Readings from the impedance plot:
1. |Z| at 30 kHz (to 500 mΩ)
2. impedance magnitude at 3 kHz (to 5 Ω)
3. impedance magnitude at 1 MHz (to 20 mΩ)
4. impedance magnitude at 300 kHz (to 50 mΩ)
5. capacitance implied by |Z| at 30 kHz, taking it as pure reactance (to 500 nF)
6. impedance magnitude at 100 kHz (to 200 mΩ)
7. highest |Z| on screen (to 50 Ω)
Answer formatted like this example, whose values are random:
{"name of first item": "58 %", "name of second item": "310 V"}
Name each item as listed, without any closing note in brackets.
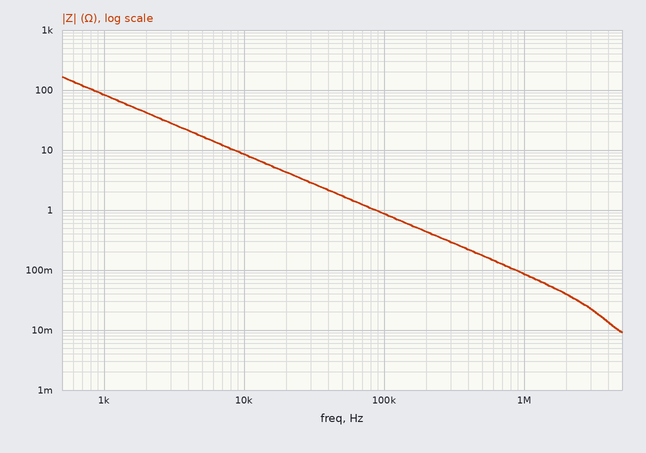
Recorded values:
{"|Z| at 30 kHz": "3.0 Ω", "impedance magnitude at 3 kHz": "30 Ω", "impedance magnitude at 1 MHz": "80 mΩ", "impedance magnitude at 300 kHz": "300 mΩ", "capacitance implied by |Z| at 30 kHz, taking it as pure reactance": "2.0 µF", "impedance magnitude at 100 kHz": "800 mΩ", "highest |Z| on screen": "150 Ω"}
